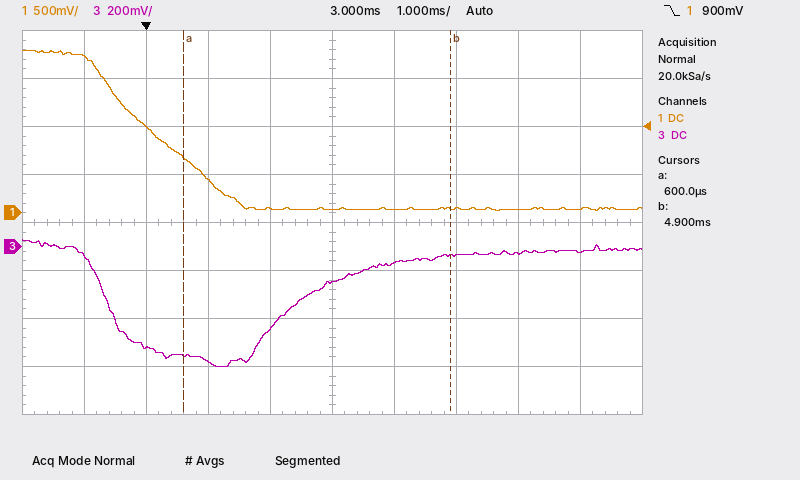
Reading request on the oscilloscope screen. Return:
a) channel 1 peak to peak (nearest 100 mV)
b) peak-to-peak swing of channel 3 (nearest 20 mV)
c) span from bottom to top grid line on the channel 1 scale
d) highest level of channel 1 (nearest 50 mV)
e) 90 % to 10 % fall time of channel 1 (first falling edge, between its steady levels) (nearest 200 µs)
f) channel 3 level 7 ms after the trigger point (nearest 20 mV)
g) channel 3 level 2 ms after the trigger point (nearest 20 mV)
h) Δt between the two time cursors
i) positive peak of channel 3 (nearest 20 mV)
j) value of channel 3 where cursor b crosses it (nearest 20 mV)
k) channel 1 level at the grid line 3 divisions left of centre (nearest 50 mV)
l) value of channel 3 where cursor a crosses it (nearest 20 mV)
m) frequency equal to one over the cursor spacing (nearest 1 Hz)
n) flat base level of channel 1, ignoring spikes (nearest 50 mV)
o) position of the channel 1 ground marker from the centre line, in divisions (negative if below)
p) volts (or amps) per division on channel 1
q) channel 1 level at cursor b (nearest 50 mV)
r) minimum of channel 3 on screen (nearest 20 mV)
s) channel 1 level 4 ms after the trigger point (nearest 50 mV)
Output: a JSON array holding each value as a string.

["1.70 V", "520 mV", "4 V", "1.70 V", "2.0 ms", "-20 mV", "-340 mV", "4.3 ms", "20 mV", "-40 mV", "900 mV", "-460 mV", "233 Hz", "50 mV", "+0.2 div", "500 mV", "50 mV", "-500 mV", "50 mV"]
